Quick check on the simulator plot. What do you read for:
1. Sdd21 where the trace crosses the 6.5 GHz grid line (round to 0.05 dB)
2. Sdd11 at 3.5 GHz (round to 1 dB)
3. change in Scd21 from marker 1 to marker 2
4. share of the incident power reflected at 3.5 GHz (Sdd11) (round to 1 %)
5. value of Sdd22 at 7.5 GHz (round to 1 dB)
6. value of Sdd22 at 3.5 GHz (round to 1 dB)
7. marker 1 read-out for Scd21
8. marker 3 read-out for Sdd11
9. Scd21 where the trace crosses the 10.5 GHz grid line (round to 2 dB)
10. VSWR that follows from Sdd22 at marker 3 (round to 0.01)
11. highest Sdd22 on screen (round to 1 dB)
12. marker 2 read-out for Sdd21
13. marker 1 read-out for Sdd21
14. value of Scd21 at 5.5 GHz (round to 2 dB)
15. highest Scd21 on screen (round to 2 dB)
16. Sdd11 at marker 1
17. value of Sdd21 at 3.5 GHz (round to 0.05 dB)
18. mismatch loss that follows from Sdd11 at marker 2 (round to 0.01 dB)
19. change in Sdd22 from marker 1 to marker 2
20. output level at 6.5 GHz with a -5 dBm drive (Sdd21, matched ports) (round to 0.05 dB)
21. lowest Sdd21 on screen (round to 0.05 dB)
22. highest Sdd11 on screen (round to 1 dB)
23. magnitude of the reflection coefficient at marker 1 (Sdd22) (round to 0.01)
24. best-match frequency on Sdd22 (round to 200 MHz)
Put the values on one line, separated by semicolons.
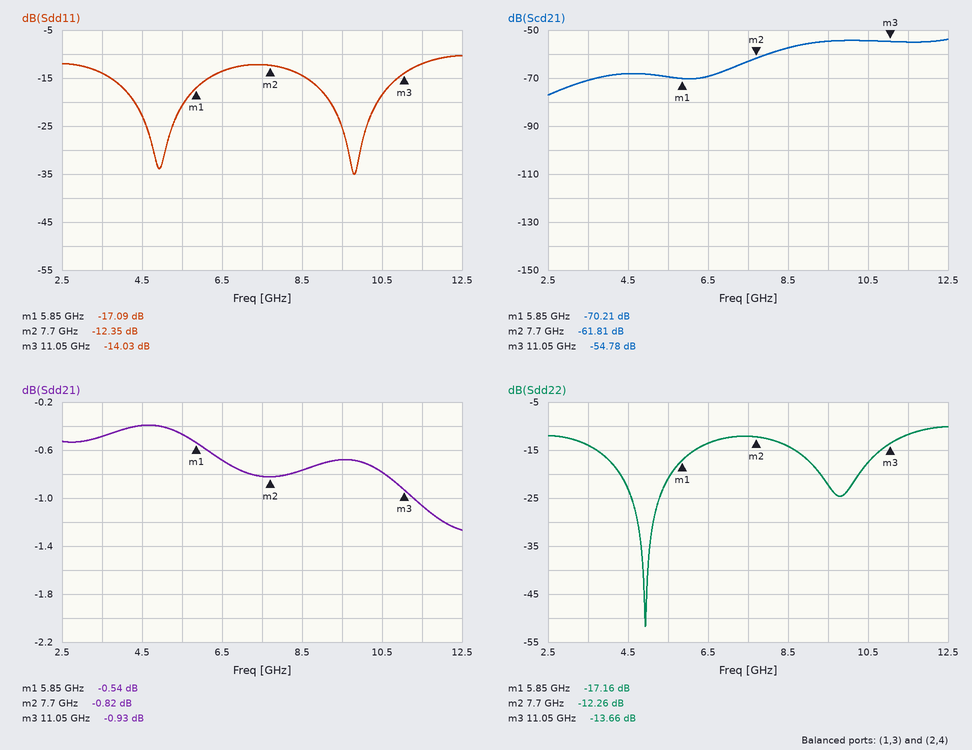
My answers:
-0.70 dB; -14 dB; 8.40 dB; 4 %; -12 dB; -14 dB; -70.21 dB; -14.03 dB; -54 dB; 1.52; -10 dB; -0.82 dB; -0.54 dB; -70 dB; -54 dB; -17.09 dB; -0.50 dB; 0.26 dB; 4.90 dB; -5.70 dBm; -1.25 dB; -10 dB; 0.14; 5.0 GHz
